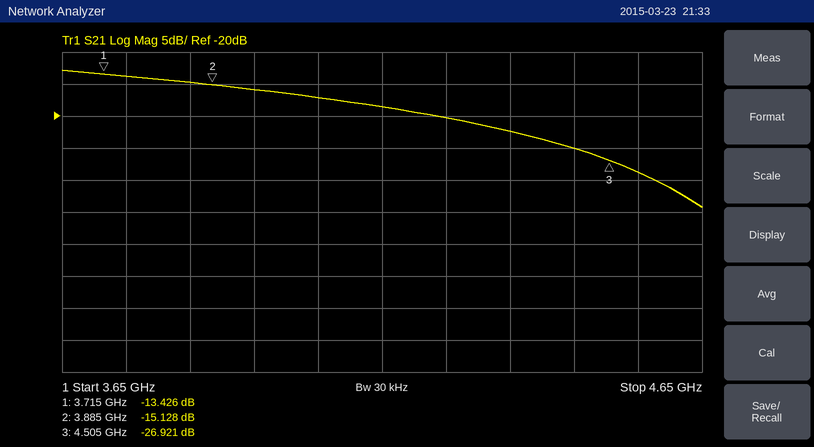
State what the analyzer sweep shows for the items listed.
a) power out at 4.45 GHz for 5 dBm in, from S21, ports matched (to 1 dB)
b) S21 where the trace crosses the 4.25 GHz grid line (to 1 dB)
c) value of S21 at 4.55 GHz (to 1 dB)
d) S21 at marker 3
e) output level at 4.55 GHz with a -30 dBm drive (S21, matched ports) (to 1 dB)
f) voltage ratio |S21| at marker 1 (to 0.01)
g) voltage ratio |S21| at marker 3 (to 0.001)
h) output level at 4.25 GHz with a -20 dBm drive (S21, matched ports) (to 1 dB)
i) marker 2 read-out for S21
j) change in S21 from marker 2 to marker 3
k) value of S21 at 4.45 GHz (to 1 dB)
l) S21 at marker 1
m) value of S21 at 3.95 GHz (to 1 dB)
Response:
-20 dBm
-20 dB
-29 dB
-26.921 dB
-59 dBm
0.21
0.045
-40 dBm
-15.128 dB
-11.793 dB
-25 dB
-13.426 dB
-16 dB
